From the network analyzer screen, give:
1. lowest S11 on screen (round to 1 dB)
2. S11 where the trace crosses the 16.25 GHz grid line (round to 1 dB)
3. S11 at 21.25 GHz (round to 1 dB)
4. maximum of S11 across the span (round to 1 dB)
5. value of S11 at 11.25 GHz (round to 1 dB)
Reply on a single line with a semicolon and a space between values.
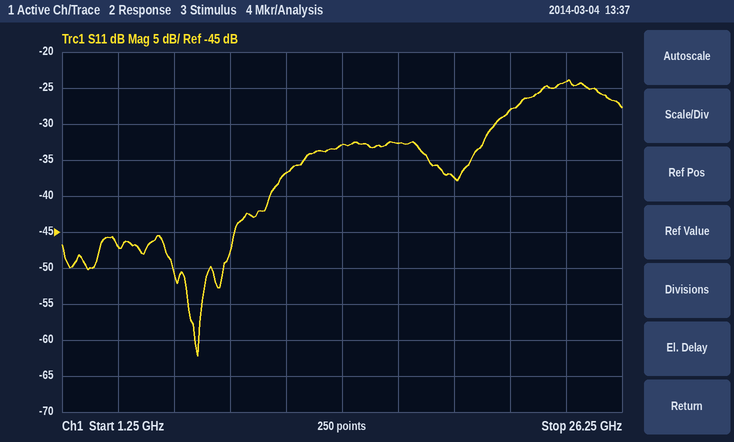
-62 dB; -33 dB; -28 dB; -24 dB; -37 dB
